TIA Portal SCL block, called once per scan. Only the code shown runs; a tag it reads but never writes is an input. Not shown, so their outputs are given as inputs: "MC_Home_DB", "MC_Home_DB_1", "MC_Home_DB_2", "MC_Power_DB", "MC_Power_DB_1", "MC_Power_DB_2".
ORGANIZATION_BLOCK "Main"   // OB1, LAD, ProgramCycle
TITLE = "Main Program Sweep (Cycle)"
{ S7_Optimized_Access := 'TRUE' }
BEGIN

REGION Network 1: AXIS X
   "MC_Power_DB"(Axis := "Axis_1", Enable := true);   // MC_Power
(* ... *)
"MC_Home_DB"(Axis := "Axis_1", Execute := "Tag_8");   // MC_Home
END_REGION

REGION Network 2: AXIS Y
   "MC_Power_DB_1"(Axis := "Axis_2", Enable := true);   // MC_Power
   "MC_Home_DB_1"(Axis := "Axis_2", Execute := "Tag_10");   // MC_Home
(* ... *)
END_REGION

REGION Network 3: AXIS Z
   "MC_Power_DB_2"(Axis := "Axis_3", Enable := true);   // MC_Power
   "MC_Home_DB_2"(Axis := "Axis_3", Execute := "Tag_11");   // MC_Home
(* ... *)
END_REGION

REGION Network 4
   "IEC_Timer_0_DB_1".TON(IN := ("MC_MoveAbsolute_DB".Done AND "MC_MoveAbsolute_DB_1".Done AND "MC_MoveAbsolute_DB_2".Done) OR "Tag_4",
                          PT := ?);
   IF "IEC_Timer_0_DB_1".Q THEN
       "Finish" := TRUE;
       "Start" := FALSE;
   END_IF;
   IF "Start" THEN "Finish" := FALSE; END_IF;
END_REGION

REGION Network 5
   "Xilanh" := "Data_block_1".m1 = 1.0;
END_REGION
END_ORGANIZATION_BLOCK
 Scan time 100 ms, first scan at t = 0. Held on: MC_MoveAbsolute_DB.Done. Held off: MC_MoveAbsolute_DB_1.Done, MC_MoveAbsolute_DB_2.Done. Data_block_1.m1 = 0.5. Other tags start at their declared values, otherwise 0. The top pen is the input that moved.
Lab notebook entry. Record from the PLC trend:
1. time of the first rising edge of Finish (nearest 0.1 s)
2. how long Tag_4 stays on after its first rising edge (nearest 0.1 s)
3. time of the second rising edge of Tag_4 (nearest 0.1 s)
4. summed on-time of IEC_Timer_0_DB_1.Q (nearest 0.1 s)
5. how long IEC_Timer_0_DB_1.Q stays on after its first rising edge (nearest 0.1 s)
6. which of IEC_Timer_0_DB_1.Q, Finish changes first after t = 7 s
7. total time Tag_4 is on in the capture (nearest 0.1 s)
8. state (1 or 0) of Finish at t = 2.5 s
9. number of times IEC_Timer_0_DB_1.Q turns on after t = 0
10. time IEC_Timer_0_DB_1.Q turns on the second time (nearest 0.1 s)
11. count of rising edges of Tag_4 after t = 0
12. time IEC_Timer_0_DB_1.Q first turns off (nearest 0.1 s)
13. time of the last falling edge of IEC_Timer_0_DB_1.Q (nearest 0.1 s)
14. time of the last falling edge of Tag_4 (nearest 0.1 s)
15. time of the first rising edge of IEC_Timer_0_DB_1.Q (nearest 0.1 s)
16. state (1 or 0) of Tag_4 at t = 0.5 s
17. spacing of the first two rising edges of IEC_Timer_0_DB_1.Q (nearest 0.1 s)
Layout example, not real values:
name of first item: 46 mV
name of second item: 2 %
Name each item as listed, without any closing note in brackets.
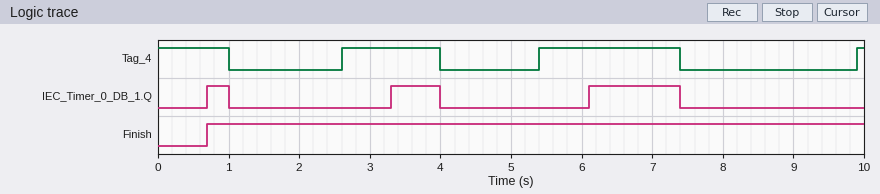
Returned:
time of the first rising edge of Finish: 0.7 s
how long Tag_4 stays on after its first rising edge: 1.4 s
time of the second rising edge of Tag_4: 5.4 s
summed on-time of IEC_Timer_0_DB_1.Q: 2.3 s
how long IEC_Timer_0_DB_1.Q stays on after its first rising edge: 0.3 s
which of IEC_Timer_0_DB_1.Q, Finish changes first after t = 7 s: IEC_Timer_0_DB_1.Q
total time Tag_4 is on in the capture: 4.5 s
state (1 or 0) of Finish at t = 2.5 s: 1
number of times IEC_Timer_0_DB_1.Q turns on after t = 0: 3
time IEC_Timer_0_DB_1.Q turns on the second time: 3.3 s
count of rising edges of Tag_4 after t = 0: 3
time IEC_Timer_0_DB_1.Q first turns off: 1.0 s
time of the last falling edge of IEC_Timer_0_DB_1.Q: 7.4 s
time of the last falling edge of Tag_4: 7.4 s
time of the first rising edge of IEC_Timer_0_DB_1.Q: 0.7 s
state (1 or 0) of Tag_4 at t = 0.5 s: 1
spacing of the first two rising edges of IEC_Timer_0_DB_1.Q: 2.6 s
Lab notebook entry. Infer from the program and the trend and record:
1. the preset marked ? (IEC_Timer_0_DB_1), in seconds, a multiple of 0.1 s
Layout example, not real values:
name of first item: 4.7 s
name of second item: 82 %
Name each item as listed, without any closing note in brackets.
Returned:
the preset marked ? (IEC_Timer_0_DB_1), in seconds, a multiple of 0.1 s: 0.7 s
